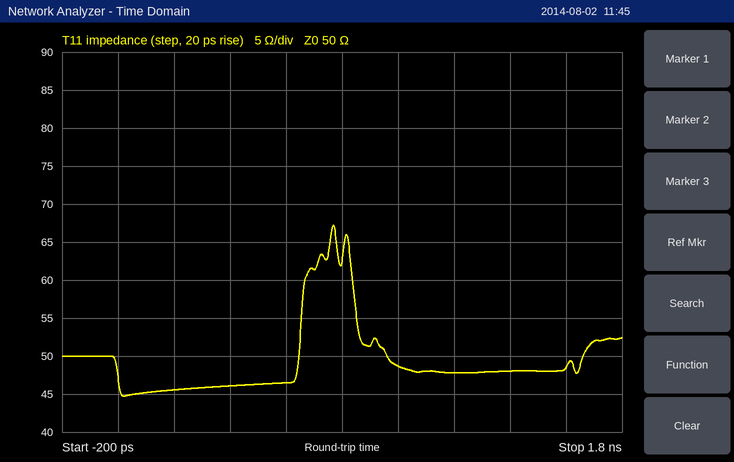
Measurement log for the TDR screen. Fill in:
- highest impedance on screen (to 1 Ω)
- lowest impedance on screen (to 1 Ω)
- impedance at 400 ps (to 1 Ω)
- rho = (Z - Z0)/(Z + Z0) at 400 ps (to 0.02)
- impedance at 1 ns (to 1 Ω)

67 Ω
45 Ω
46 Ω
-0.04
49 Ω
